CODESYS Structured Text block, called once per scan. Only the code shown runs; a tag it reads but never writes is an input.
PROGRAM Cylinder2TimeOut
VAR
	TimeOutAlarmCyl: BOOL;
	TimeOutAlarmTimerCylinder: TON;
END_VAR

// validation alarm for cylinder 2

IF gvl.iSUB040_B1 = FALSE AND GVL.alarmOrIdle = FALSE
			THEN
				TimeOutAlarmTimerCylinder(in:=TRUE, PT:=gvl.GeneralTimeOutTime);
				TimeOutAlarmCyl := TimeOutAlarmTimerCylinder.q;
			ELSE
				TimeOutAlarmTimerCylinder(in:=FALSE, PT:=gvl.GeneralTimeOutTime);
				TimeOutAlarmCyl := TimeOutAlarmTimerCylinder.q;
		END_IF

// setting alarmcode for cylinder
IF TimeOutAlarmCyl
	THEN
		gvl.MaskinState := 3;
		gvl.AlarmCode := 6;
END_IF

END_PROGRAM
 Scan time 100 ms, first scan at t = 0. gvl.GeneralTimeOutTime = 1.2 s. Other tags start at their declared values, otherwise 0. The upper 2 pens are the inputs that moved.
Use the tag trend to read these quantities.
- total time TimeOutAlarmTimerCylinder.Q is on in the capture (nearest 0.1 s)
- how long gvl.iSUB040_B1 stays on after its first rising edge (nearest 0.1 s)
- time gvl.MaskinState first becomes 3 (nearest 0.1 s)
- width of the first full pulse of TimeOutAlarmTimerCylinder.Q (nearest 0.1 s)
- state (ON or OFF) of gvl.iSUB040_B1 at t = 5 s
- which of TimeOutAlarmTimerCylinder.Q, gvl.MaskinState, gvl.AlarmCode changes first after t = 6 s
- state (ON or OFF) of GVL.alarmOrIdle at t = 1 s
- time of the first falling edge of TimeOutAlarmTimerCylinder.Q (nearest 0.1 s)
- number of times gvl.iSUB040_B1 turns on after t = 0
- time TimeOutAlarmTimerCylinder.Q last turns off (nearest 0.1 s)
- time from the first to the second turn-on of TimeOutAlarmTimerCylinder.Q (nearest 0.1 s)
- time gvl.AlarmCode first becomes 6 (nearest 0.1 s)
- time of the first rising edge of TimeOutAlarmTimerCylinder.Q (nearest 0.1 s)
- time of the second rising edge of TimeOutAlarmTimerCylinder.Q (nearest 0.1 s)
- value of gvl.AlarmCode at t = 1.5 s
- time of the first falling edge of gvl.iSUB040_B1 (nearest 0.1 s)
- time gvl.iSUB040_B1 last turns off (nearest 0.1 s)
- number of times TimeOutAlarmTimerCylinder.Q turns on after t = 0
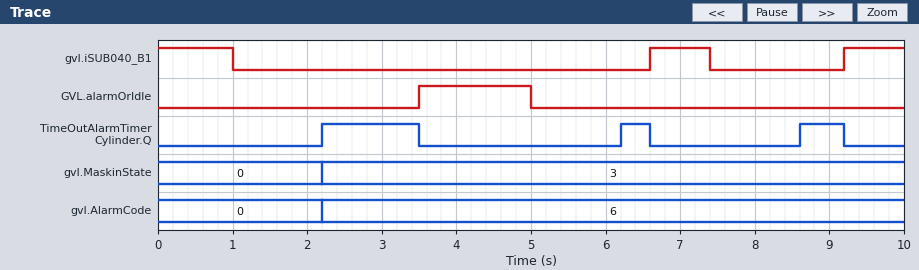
2.3 s
0.8 s
2.2 s
1.3 s
OFF
TimeOutAlarmTimerCylinder.Q
OFF
3.5 s
2
9.2 s
4.0 s
2.2 s
2.2 s
6.2 s
0
1.0 s
7.4 s
3
